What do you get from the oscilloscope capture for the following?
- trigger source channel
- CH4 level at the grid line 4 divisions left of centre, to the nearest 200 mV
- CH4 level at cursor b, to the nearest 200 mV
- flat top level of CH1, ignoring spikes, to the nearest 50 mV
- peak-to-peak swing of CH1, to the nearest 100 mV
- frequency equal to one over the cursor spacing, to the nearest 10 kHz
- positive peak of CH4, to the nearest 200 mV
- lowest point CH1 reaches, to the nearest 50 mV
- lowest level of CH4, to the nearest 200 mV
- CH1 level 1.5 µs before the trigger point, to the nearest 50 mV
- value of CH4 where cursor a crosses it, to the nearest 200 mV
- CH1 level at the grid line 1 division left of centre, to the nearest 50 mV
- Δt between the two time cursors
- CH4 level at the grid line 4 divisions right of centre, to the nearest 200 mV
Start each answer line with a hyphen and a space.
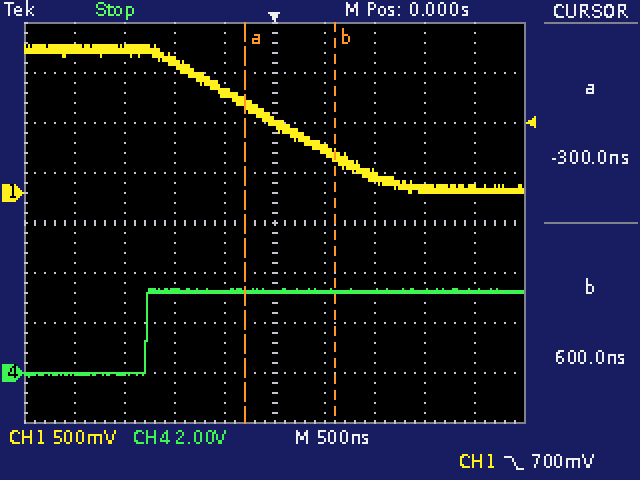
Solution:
- CH1
- 0.0 V
- 3.2 V
- 1.45 V
- 1.50 V
- 1.11 MHz
- 3.4 V
- 0 mV
- -200 mV
- 1.45 V
- 3.2 V
- 1.00 V
- 900 ns
- 3.2 V
